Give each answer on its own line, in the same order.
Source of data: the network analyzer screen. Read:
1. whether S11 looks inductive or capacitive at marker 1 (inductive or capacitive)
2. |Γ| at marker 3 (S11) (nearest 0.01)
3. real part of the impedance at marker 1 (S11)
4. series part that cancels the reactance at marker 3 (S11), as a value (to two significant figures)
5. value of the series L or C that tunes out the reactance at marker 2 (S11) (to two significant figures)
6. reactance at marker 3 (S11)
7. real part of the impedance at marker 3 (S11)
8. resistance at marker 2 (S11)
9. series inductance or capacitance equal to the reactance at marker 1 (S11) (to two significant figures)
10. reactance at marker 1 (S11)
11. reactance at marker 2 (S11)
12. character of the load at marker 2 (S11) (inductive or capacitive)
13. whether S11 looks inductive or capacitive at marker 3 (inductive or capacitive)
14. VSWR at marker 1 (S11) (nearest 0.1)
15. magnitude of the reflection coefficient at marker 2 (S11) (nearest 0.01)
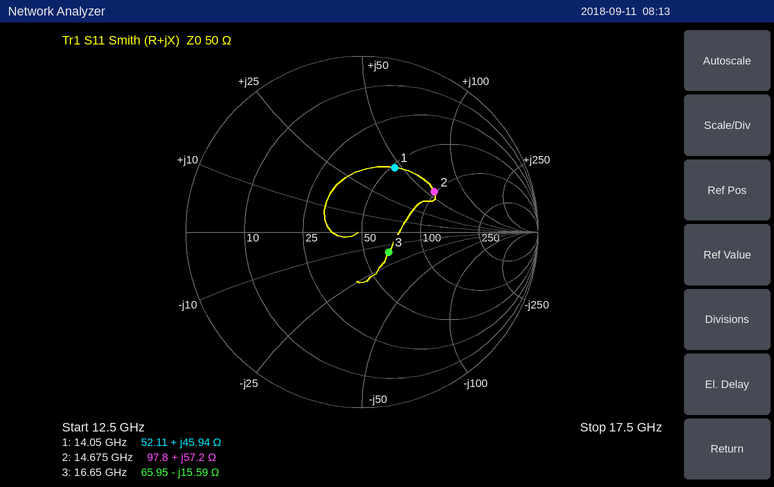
inductive
0.19
52.11 Ω
150 pH
190 fF
-15.59 Ω
65.95 Ω
97.8 Ω
520 pH
+45.94 Ω
+57.2 Ω
inductive
capacitive
2.4
0.47
